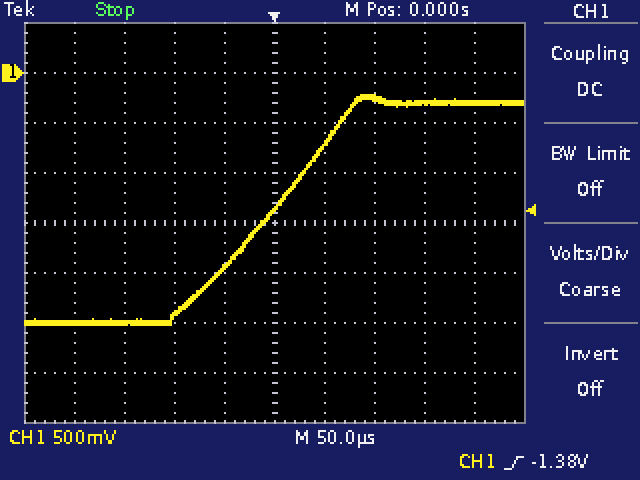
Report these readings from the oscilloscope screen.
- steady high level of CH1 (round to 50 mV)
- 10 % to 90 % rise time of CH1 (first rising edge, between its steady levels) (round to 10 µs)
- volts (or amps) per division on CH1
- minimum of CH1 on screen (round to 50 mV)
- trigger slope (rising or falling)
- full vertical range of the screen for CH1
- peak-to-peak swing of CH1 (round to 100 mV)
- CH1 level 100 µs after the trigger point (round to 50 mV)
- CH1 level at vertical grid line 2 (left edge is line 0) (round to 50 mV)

-300 mV
150 µs
500 mV
-2.50 V
rising
4 V
2.30 V
-250 mV
-2.50 V
